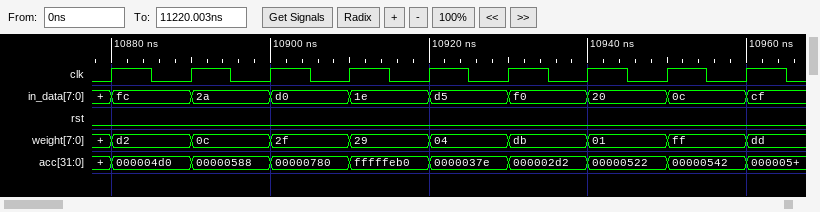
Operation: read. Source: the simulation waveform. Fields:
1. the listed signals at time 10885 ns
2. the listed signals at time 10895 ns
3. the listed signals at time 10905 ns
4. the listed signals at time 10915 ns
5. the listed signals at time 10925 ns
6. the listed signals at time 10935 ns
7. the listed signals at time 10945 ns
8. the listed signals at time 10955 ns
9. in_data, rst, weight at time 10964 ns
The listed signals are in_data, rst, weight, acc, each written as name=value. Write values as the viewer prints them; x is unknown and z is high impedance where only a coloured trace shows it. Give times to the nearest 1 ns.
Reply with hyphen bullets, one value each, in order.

- in_data=fc, rst=0, weight=d2, acc=000004d0
- in_data=2a, rst=0, weight=0c, acc=00000588
- in_data=d0, rst=0, weight=2f, acc=00000780
- in_data=1e, rst=0, weight=29, acc=fffffeb0
- in_data=d5, rst=0, weight=04, acc=0000037e
- in_data=f0, rst=0, weight=db, acc=000002d2
- in_data=20, rst=0, weight=01, acc=00000522
- in_data=0c, rst=0, weight=ff, acc=00000542
- in_data=cf, rst=0, weight=dd
